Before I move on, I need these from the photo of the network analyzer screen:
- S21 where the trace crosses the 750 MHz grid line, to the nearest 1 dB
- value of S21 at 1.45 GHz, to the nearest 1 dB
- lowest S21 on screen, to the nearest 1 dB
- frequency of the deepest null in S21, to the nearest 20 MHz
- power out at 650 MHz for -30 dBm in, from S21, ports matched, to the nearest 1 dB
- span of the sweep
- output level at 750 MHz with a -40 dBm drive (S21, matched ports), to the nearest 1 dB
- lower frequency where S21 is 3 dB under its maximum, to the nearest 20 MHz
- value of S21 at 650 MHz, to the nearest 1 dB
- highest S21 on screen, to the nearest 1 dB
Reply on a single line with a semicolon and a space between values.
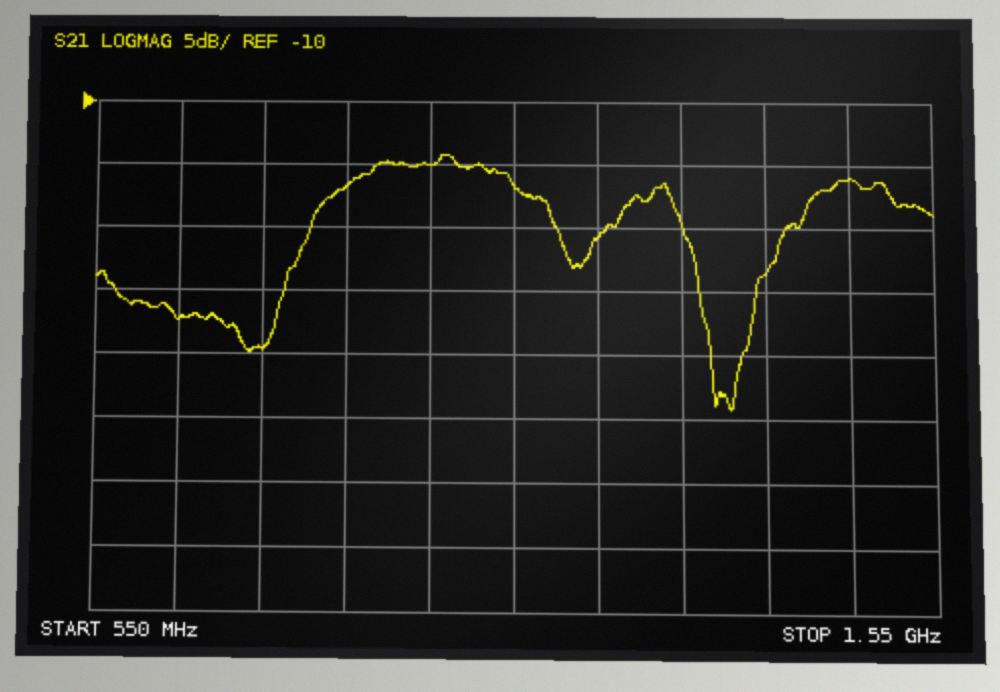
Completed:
-30 dB; -16 dB; -34 dB; 1.30 GHz; -57 dBm; 1 GHz; -70 dBm; 840 MHz; -27 dB; -14 dB
